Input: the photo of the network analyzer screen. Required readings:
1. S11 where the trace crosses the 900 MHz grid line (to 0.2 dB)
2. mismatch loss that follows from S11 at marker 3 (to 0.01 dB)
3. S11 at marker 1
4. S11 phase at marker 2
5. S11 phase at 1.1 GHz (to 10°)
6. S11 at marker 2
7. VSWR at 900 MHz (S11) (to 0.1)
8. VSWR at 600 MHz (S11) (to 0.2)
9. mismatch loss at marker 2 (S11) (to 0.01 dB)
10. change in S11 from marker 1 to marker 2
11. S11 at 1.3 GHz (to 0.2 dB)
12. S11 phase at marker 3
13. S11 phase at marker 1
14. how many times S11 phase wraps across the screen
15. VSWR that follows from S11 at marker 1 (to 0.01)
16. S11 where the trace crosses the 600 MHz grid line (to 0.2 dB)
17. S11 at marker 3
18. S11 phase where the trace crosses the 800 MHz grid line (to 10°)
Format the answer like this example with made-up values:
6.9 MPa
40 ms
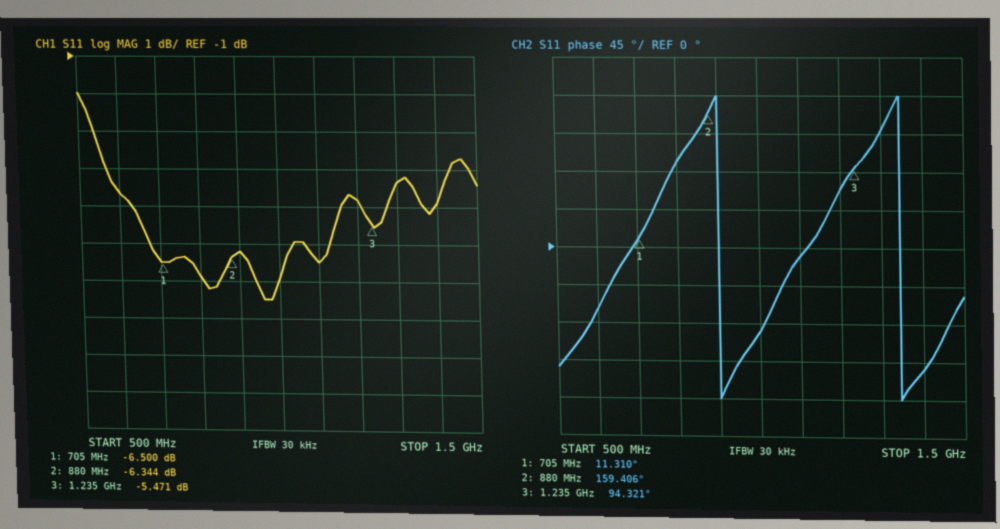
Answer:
-6.2 dB
1.45 dB
-6.500 dB
159.406°
-10°
-6.344 dB
2.9
3.8
1.15 dB
0.156 dB
-4.4 dB
94.321°
11.310°
2
2.80
-4.6 dB
-5.471 dB
100°
